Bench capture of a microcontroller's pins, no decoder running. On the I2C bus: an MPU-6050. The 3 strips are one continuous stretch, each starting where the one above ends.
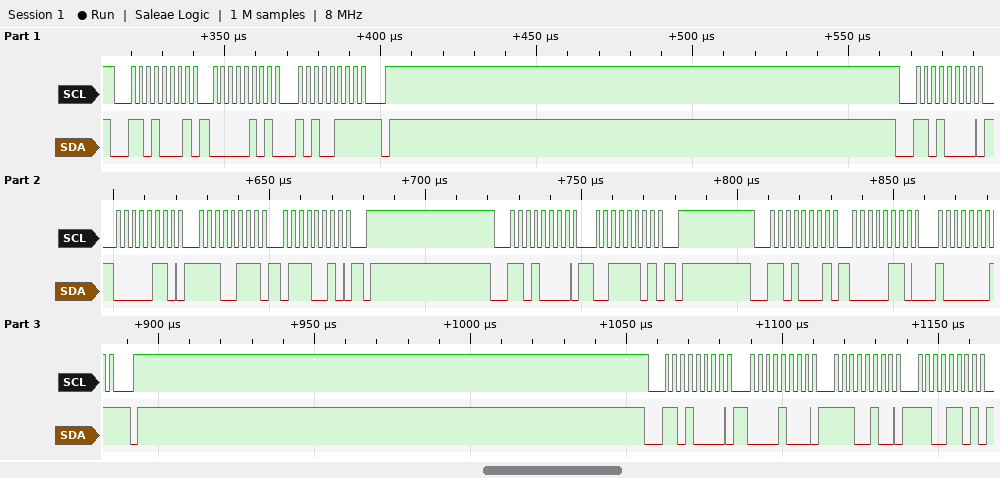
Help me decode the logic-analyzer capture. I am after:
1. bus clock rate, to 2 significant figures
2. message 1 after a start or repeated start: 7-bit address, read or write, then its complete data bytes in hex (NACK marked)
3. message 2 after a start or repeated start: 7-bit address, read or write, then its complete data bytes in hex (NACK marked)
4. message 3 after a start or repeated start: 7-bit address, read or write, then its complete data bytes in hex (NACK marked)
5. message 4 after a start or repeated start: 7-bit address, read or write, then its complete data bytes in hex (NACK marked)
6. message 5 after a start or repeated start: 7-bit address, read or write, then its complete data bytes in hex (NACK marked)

400 kHz
0x68 read: 05 A7 NACK
0x68 write: 06 E7 72
0x68 write: 3D
0x68 read: 06 81 NACK
0x68 write: 08 E4 CD
